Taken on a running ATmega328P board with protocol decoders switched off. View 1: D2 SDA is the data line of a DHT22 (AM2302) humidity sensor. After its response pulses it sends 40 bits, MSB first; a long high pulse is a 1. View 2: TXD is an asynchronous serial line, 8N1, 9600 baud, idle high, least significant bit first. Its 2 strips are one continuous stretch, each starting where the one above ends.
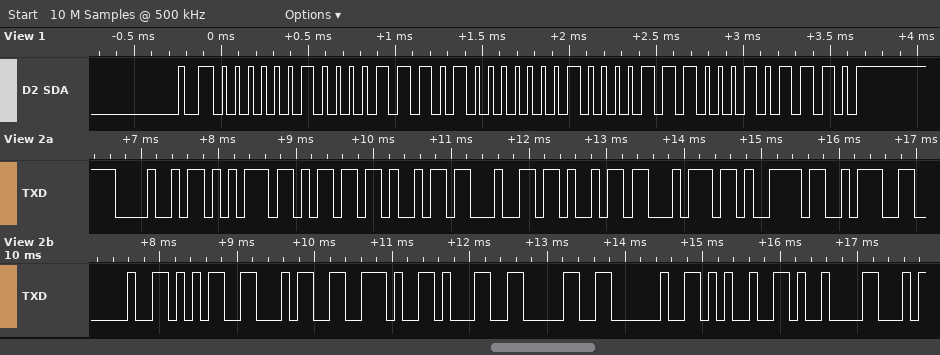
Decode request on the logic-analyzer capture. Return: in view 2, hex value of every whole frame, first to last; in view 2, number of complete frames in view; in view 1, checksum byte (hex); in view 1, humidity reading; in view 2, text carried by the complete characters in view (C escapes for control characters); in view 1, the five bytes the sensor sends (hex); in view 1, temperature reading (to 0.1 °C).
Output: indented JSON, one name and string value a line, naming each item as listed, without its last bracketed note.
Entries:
{
  "in view 2, hex value of every whole frame, first to last": "48 75 6D 69 64 69 74 79 3A 20 35 34 2E 31 30 20 25 09",
  "in view 2, number of complete frames in view": "18",
  "in view 1, checksum byte": "0x2E",
  "in view 1, humidity reading": "54.1 %",
  "in view 2, text carried by the complete characters in view": "\"Humidity: 54.10 %\\t\"",
  "in view 1, the five bytes the sensor sends": "02 1D 01 0E 2E",
  "in view 1, temperature reading": "27.0 °C"
}
